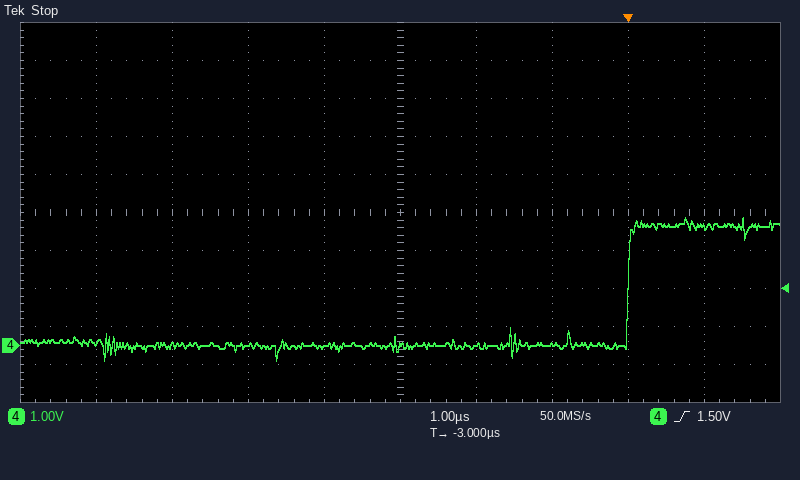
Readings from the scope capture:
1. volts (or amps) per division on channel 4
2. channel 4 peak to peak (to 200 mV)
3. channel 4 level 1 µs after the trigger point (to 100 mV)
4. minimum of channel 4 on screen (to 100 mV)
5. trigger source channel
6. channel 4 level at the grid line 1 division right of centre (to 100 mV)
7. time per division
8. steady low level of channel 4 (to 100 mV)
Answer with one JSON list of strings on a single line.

["1 V", "3.8 V", "3.1 V", "-400 mV", "channel 4", "0.0 V", "1 µs", "0.0 V"]
